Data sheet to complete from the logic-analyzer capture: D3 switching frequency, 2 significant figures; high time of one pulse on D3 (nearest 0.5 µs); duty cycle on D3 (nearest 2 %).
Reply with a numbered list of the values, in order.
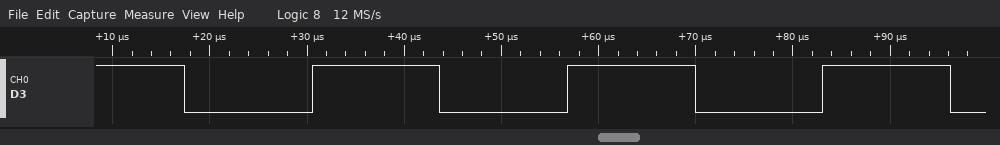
1. 38 kHz
2. 13.0 µs
3. 50 %
